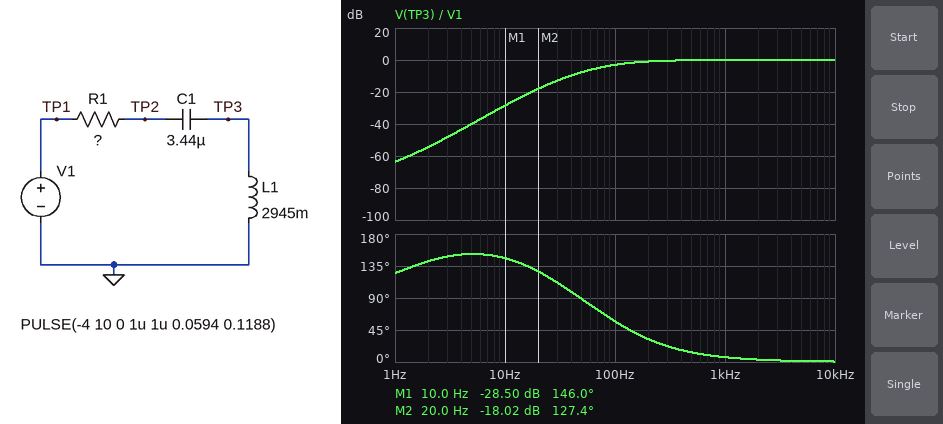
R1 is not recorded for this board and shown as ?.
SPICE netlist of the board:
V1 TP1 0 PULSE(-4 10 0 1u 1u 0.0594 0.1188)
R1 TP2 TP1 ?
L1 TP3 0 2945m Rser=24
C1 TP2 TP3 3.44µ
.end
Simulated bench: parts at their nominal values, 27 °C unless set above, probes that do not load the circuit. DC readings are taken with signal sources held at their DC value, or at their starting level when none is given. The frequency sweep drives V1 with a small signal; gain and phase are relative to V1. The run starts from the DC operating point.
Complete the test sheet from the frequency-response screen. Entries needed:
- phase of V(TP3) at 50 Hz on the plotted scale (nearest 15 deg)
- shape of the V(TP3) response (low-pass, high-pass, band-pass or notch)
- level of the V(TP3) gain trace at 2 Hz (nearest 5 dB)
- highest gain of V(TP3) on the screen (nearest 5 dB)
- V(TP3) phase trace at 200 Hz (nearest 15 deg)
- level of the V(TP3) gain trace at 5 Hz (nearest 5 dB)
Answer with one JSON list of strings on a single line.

["90 deg", "high-pass", "-55 dB", "0 dB", "30 deg", "-40 dB"]
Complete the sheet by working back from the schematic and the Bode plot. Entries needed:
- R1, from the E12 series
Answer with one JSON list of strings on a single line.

["2.2 kΩ"]
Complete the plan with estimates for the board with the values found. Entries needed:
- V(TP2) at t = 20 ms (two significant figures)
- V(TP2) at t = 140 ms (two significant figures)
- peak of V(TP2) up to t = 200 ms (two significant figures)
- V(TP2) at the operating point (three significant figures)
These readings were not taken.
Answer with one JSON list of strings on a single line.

["9.1 V", "9.3 V", "10 V", "-4.00 V"]
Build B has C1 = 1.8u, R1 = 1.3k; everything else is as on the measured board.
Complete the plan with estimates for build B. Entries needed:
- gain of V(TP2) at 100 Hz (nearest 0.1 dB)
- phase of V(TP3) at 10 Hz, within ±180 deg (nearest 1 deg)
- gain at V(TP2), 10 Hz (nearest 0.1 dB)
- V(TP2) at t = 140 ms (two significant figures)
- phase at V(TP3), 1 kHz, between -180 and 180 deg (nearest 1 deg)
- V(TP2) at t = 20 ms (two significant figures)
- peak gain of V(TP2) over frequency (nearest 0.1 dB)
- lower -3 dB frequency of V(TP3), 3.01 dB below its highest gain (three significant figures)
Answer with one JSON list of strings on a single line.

["-4.6 dB", "164 deg", "-0.1 dB", "9.9 V", "4 deg", "9.8 V", "0 dB", "59.5 Hz"]
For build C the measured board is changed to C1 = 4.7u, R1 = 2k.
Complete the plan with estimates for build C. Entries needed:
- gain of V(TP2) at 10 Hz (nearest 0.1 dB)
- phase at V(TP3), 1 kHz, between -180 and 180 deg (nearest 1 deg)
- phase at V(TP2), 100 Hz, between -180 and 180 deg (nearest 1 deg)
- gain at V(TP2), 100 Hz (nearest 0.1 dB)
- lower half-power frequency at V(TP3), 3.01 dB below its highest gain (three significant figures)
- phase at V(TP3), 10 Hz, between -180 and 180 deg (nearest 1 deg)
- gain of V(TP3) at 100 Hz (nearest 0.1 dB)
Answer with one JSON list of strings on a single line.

["-1.5 dB", "6 deg", "52 deg", "-4.5 dB", "93.2 Hz", "140 deg", "-2.7 dB"]
